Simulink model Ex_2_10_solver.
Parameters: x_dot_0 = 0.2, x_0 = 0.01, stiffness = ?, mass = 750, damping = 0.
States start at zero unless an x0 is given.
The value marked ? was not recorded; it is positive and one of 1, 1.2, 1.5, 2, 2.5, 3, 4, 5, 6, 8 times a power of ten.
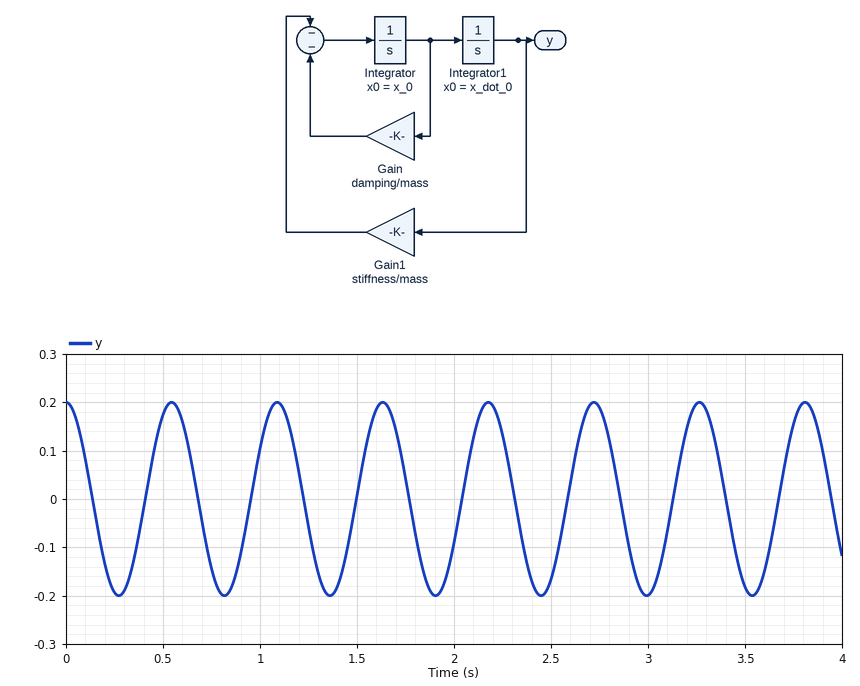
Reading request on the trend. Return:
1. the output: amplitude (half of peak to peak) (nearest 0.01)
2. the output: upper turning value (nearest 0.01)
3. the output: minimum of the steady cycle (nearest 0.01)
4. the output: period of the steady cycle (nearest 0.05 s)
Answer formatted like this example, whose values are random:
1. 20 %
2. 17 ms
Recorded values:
1. 0.20
2. 0.20
3. -0.20
4. 0.55 s
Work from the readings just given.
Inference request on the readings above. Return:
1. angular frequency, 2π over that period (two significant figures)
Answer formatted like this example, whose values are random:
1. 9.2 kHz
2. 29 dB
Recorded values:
1. 11 rad/s
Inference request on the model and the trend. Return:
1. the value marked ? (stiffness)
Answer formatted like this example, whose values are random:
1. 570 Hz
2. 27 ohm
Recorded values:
1. 100000
